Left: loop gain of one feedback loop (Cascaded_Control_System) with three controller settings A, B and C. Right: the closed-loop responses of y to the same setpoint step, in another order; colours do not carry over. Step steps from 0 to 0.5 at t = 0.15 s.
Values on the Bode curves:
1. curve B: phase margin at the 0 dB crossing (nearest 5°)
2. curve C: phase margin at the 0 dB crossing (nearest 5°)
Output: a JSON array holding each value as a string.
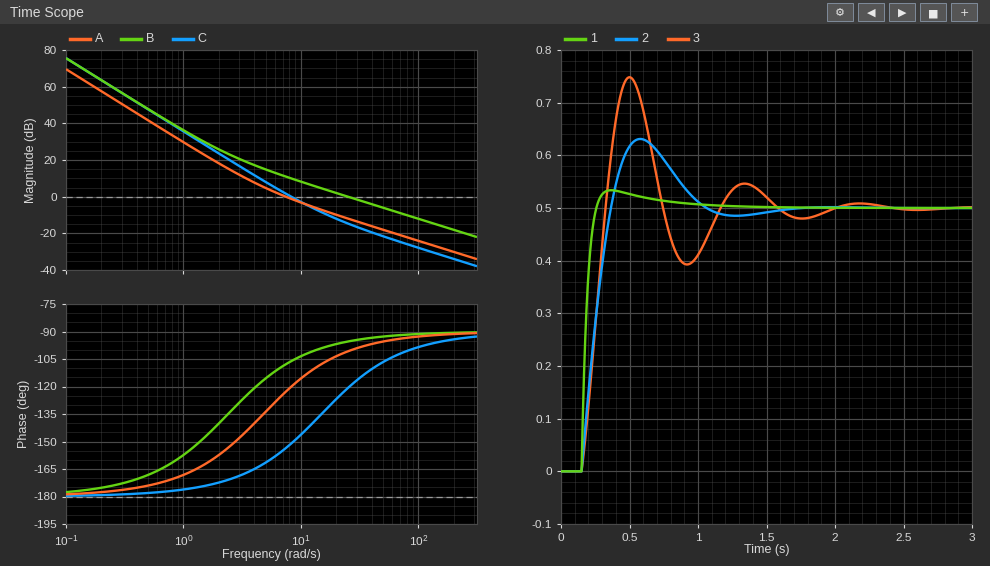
["85°", "30°"]
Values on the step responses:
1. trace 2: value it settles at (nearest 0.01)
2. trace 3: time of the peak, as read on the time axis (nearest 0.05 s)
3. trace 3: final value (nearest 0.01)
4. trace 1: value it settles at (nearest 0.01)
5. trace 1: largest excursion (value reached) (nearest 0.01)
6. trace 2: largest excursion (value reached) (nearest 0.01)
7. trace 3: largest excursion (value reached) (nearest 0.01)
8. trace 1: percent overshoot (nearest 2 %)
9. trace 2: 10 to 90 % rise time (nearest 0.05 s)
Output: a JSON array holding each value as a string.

["0.50", "0.50 s", "0.50", "0.50", "0.53", "0.63", "0.75", "6 %", "0.15 s"]
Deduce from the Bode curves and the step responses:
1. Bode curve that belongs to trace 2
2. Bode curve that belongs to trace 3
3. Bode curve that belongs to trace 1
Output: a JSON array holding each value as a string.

["A", "C", "B"]
